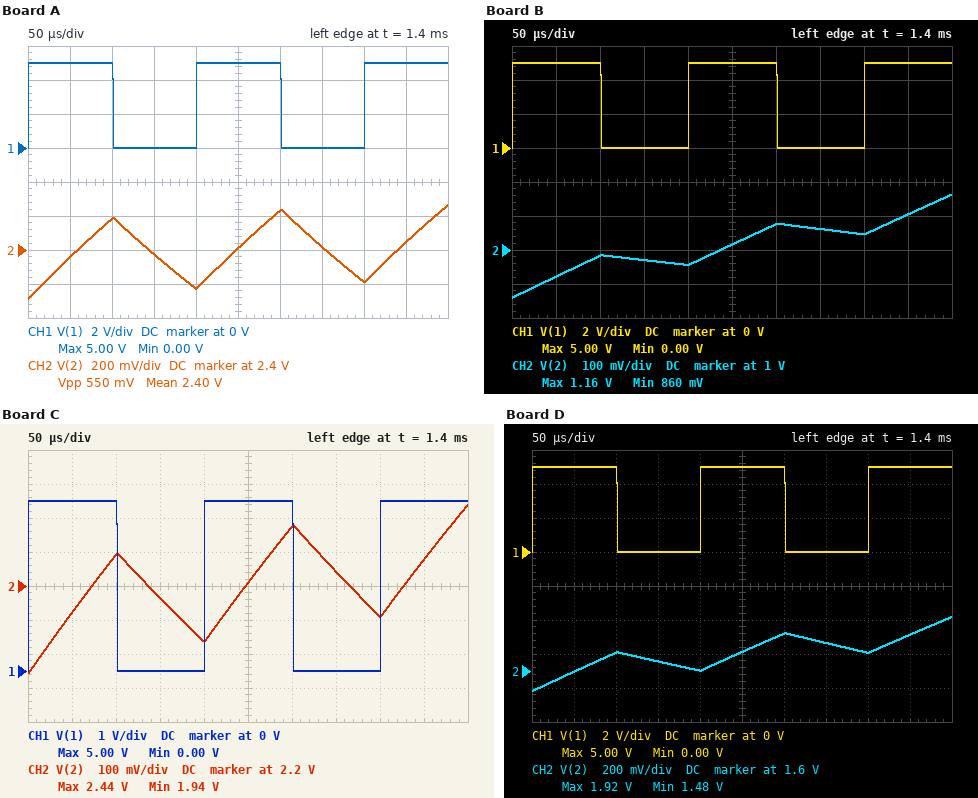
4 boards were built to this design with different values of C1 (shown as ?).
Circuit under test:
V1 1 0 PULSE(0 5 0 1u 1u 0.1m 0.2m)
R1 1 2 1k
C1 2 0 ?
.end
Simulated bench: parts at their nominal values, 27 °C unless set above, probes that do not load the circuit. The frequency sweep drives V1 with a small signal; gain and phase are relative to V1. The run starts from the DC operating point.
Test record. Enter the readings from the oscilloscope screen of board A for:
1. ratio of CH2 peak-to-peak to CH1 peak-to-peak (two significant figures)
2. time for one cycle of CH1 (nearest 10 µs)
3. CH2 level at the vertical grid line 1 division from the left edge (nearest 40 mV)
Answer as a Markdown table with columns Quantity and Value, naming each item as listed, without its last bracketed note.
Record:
| Quantity | Value |
|---|---|
| ratio of CH2 peak-to-peak to CH1 peak-to-peak | 0.11 |
| time for one cycle of CH1 | 200 µs |
| CH2 level at the vertical grid line 1 division from the left edge | 2.36 V |
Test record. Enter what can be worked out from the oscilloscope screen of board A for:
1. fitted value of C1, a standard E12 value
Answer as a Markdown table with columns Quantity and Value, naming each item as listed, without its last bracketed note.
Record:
| Quantity | Value |
|---|---|
| fitted value of C1, a standard E12 value | 560 nF |
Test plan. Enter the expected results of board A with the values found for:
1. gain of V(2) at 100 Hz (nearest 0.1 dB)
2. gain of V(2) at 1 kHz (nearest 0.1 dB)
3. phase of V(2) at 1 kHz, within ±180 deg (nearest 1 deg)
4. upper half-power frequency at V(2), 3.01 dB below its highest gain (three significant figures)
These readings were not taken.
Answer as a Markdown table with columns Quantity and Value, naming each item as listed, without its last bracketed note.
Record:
| Quantity | Value |
|---|---|
| gain of V(2) at 100 Hz | -0.5 dB |
| gain of V(2) at 1 kHz | -11.3 dB |
| phase of V(2) at 1 kHz, within ±180 deg | -74 deg |
| upper half-power frequency at V(2), 3.01 dB below its highest gain | 284 Hz |
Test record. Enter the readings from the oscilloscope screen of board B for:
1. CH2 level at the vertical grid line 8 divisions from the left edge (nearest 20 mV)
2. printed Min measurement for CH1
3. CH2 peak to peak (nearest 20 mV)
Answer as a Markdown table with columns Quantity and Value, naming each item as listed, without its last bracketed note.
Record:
| Quantity | Value |
|---|---|
| CH2 level at the vertical grid line 8 divisions from the left edge | 1.04 V |
| printed Min measurement for CH1 | 0.00 V |
| CH2 peak to peak | 300 mV |
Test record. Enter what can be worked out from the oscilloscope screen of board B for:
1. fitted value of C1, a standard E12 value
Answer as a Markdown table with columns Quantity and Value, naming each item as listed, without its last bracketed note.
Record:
| Quantity | Value |
|---|---|
| fitted value of C1, a standard E12 value | 3.3 µF |
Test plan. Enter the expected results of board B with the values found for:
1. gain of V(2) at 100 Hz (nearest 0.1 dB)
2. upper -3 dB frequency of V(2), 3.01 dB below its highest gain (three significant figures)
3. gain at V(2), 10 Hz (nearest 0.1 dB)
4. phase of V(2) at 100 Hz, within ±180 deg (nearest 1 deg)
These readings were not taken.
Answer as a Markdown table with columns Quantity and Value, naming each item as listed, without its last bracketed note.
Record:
| Quantity | Value |
|---|---|
| gain of V(2) at 100 Hz | -7.2 dB |
| upper -3 dB frequency of V(2), 3.01 dB below its highest gain | 48.2 Hz |
| gain at V(2), 10 Hz | -0.2 dB |
| phase of V(2) at 100 Hz, within ±180 deg | -64 deg |
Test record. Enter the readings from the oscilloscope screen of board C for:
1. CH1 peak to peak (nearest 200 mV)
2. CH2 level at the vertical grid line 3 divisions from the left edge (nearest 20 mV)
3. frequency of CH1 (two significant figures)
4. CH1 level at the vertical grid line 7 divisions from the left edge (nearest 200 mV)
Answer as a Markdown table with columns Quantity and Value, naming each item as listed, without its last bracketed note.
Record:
| Quantity | Value |
|---|---|
| CH1 peak to peak | 5.0 V |
| CH2 level at the vertical grid line 3 divisions from the left edge | 2.16 V |
| frequency of CH1 | 5.0 kHz |
| CH1 level at the vertical grid line 7 divisions from the left edge | 0 V |
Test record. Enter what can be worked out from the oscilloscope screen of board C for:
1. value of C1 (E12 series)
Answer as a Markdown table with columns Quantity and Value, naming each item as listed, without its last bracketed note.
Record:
| Quantity | Value |
|---|---|
| value of C1 | 820 nF |
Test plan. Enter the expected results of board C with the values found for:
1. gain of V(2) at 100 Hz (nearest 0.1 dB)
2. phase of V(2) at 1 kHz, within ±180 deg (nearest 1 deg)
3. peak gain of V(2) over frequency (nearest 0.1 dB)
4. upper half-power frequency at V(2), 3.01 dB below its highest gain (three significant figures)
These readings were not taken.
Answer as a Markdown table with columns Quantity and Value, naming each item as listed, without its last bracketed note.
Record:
| Quantity | Value |
|---|---|
| gain of V(2) at 100 Hz | -1.0 dB |
| phase of V(2) at 1 kHz, within ±180 deg | -79 deg |
| peak gain of V(2) over frequency | 0 dB |
| upper half-power frequency at V(2), 3.01 dB below its highest gain | 194 Hz |
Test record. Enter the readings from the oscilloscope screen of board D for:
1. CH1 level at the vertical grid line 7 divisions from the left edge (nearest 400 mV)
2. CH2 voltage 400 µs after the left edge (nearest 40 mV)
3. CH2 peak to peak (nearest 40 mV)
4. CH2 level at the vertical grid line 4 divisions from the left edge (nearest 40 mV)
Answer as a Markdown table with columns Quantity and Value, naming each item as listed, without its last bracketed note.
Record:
| Quantity | Value |
|---|---|
| CH1 level at the vertical grid line 7 divisions from the left edge | 0 V |
| CH2 voltage 400 µs after the left edge | 1.72 V |
| CH2 peak to peak | 440 mV |
| CH2 level at the vertical grid line 4 divisions from the left edge | 1.60 V |
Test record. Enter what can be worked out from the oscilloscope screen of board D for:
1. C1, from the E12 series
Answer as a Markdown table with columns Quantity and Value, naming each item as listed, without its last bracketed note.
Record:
| Quantity | Value |
|---|---|
| C1, from the E12 series | 1.5 µF |
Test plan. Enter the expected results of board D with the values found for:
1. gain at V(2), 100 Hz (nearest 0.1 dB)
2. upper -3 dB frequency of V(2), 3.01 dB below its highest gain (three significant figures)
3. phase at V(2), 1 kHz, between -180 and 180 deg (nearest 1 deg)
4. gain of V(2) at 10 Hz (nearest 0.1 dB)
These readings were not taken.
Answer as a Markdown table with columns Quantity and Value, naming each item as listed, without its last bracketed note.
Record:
| Quantity | Value |
|---|---|
| gain at V(2), 100 Hz | -2.8 dB |
| upper -3 dB frequency of V(2), 3.01 dB below its highest gain | 106 Hz |
| phase at V(2), 1 kHz, between -180 and 180 deg | -84 deg |
| gain of V(2) at 10 Hz | 0 dB |
